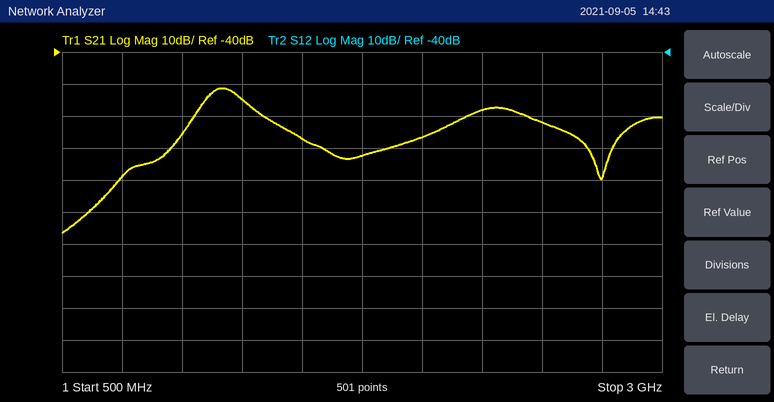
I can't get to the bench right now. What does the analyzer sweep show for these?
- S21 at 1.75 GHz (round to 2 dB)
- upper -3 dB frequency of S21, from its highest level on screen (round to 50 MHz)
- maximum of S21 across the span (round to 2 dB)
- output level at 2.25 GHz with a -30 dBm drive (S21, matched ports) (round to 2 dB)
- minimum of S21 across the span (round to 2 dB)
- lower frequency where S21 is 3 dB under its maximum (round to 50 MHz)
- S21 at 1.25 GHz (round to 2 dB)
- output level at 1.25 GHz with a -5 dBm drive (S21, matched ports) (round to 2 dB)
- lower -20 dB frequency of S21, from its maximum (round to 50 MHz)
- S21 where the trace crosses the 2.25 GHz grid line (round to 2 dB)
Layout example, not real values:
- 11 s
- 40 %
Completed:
- -72 dB
- 1.25 GHz
- -52 dB
- -88 dBm
- -96 dB
- 1.10 GHz
- -54 dB
- -60 dBm
- 950 MHz
- -58 dB
